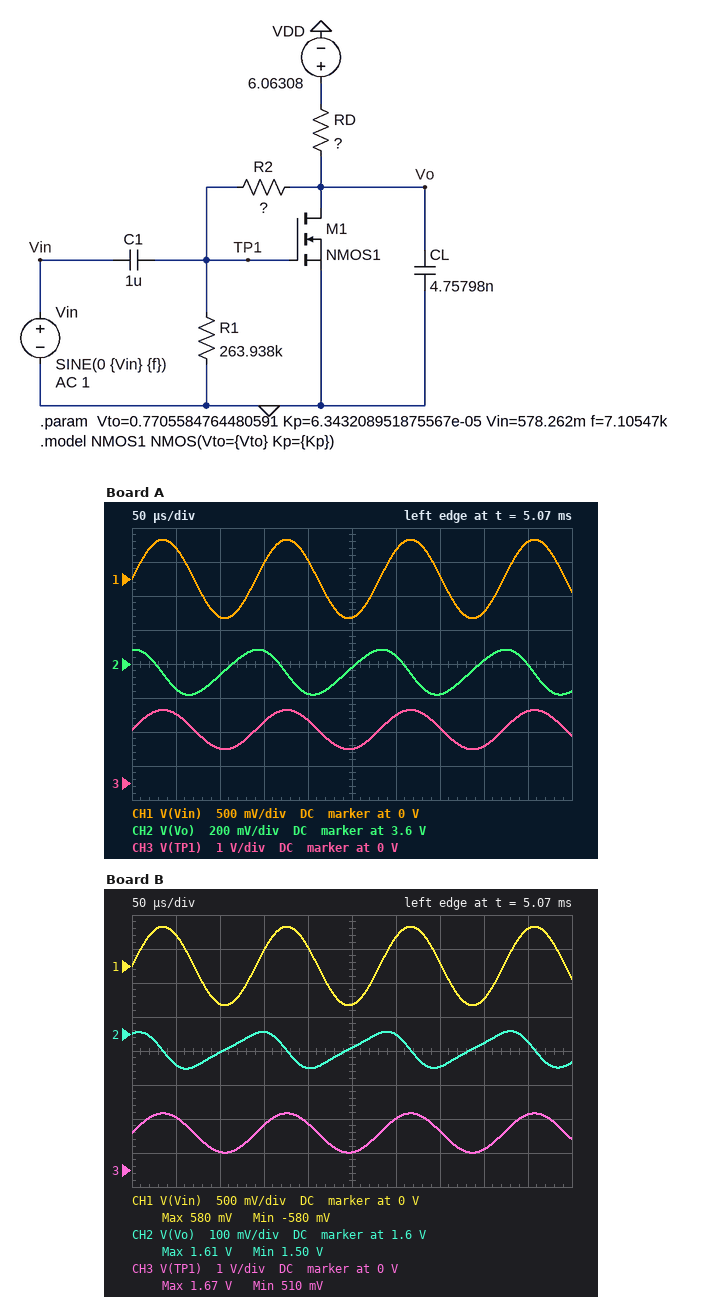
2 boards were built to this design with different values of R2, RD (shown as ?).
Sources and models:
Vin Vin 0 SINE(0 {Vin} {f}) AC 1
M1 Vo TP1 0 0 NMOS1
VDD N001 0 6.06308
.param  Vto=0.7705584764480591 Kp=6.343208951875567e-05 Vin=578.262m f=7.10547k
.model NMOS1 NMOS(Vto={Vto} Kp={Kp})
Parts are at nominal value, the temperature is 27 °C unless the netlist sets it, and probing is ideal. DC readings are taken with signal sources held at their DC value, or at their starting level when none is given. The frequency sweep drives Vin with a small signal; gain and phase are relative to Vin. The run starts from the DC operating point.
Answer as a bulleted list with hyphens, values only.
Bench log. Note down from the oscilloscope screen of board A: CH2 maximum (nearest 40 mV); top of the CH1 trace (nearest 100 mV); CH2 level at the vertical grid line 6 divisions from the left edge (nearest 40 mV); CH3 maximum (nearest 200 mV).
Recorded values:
- 3.68 V
- 600 mV
- 3.64 V
- 2.2 V
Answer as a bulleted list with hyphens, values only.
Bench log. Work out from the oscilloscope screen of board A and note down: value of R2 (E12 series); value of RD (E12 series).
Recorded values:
- 390 kΩ
- 82 kΩ
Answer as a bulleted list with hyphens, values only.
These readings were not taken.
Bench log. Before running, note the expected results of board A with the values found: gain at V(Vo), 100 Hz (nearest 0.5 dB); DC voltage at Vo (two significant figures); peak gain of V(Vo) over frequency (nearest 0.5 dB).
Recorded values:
- 10.0 dB
- 3.9 V
- 10.5 dB
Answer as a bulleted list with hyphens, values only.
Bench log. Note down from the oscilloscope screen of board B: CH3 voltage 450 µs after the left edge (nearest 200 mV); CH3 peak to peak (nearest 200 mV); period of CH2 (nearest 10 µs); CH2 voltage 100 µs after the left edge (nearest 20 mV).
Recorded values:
- 1.6 V
- 1.2 V
- 140 µs
- 1.54 V
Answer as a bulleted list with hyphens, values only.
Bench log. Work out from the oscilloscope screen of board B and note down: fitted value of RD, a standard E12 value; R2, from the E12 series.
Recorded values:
- 470 kΩ
- 330 kΩ
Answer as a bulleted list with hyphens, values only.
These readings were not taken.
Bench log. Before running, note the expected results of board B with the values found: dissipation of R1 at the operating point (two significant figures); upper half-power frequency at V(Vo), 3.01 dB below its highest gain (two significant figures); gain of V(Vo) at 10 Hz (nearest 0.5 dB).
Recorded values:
- 4.6 µW
- 180 Hz
- 10.5 dB
